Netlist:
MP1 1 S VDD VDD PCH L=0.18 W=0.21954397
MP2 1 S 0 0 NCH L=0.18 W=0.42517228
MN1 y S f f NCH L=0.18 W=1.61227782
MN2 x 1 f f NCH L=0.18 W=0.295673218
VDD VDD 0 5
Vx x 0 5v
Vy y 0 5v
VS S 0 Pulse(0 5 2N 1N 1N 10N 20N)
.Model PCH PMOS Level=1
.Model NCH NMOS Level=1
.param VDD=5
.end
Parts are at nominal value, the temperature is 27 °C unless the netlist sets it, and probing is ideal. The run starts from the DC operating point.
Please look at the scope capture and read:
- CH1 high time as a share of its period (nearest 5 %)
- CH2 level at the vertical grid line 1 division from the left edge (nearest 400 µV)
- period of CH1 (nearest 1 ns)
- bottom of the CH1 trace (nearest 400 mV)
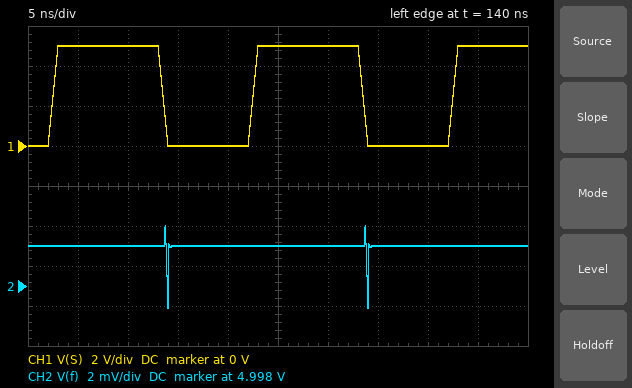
55 %
5.0000 V
20 ns
0 V
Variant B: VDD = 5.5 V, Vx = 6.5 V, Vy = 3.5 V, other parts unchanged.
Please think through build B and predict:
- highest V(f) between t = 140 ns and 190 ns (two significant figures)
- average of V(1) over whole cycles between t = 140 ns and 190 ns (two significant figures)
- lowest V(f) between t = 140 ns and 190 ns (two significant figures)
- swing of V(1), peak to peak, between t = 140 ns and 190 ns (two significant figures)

4.1 V
2.5 V
3.5 V
5.5 V
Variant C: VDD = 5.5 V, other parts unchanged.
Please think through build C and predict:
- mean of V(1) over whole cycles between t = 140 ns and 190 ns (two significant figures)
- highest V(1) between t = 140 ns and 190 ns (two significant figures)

2.5 V
5.5 V
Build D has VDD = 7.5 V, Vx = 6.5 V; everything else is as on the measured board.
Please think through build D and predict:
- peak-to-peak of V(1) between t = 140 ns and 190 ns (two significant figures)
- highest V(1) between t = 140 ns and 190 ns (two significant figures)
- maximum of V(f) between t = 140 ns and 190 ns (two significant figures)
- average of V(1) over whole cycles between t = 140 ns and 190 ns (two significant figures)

7.2 V
7.5 V
5.6 V
3.6 V
